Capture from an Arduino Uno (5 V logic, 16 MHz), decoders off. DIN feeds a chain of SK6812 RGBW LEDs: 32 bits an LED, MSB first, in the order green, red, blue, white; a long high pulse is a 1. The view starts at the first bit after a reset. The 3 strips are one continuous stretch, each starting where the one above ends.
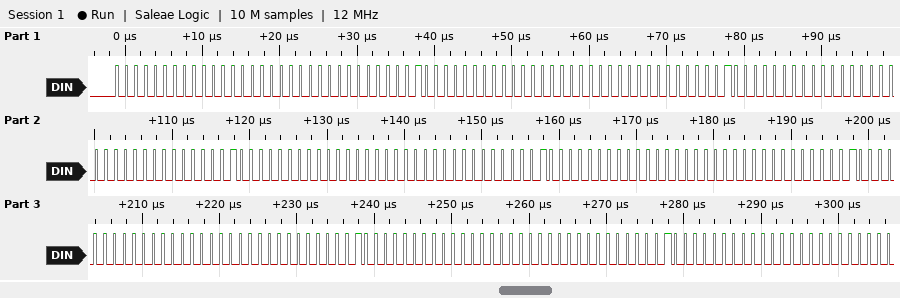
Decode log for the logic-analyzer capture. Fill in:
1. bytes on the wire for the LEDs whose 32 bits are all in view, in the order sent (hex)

00 00 00 01 00 00 00 01 00 00 00 01 00 00 00 01 00 00 00 01 00 00 00 01 00 00 00 01
